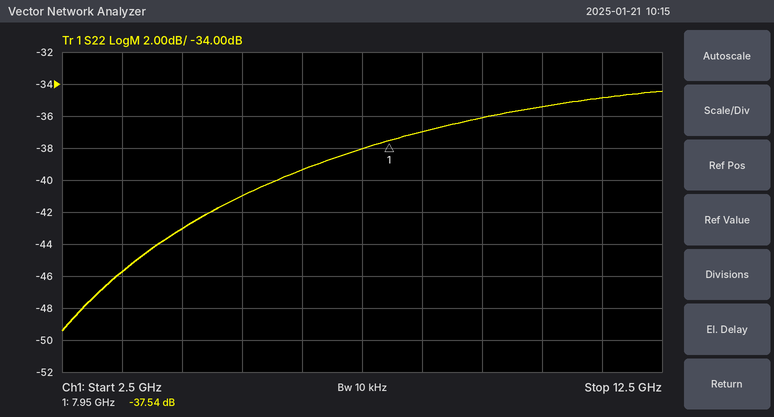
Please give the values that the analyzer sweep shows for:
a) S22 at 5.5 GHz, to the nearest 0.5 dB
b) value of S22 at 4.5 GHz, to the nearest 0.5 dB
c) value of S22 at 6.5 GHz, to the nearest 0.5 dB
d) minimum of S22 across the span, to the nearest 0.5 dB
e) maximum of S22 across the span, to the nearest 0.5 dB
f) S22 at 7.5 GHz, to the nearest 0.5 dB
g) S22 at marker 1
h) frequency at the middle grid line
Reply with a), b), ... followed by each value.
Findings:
a) -41.0 dB
b) -43.0 dB
c) -39.5 dB
d) -49.5 dB
e) -34.5 dB
f) -38.0 dB
g) -37.54 dB
h) 7.5 GHz
